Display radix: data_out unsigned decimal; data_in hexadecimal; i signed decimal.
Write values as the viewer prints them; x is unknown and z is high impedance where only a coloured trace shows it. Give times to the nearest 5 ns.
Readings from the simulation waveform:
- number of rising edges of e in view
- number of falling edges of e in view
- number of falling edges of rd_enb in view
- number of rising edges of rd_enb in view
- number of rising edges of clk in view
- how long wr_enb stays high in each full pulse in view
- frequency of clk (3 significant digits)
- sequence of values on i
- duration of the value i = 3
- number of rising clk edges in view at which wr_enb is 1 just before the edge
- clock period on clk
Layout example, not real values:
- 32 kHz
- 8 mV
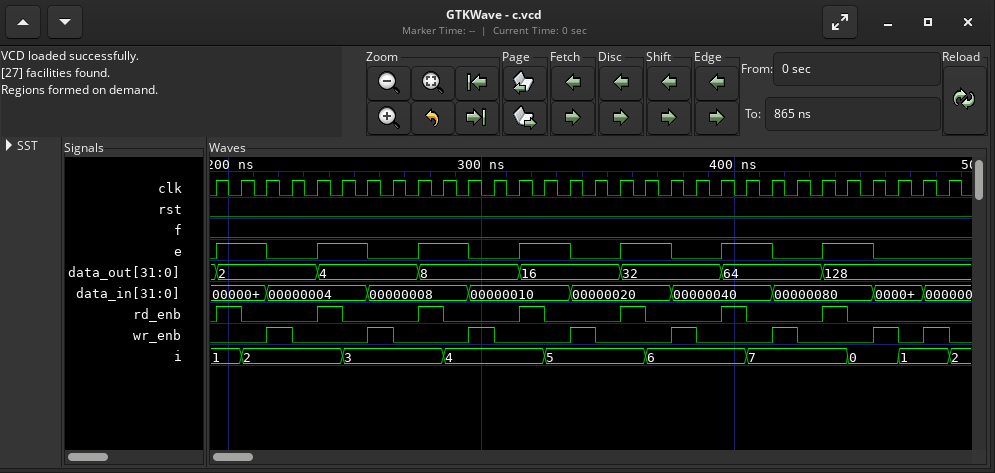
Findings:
- 7
- 7
- 7
- 7
- 30
- 10 ns, 10 ns, 10 ns, 10 ns, 10 ns, 10 ns, 10 ns, 10 ns
- 100 MHz
- 1, 2, 3, 4, 5, 6, 7, 0, 1, 2
- 40 ns
- 8
- 10 ns
